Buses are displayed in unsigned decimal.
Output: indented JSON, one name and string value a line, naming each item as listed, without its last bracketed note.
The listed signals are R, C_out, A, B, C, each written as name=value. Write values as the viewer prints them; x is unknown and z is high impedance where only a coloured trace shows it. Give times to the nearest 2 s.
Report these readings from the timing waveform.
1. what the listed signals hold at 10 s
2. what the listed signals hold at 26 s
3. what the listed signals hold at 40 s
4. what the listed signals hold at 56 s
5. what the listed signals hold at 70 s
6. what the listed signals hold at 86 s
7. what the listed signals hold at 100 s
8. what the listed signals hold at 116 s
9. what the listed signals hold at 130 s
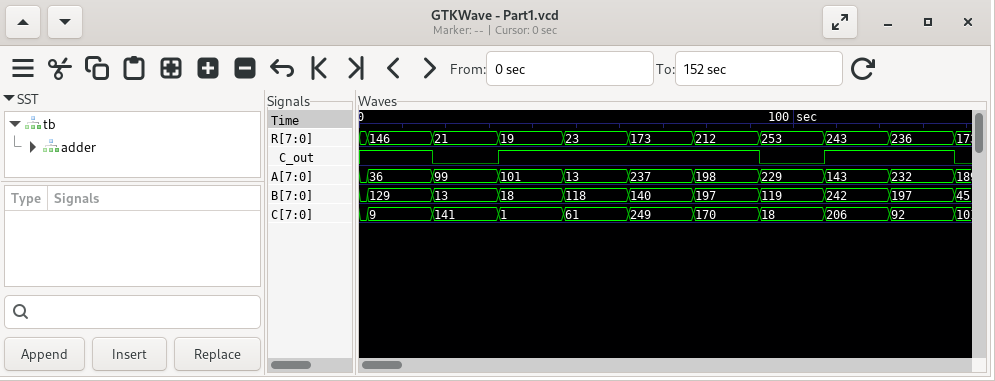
{
  "what the listed signals hold at 10 s": "R=146, C_out=1, A=36, B=129, C=9",
  "what the listed signals hold at 26 s": "R=21, C_out=0, A=99, B=13, C=141",
  "what the listed signals hold at 40 s": "R=19, C_out=1, A=101, B=18, C=1",
  "what the listed signals hold at 56 s": "R=23, C_out=1, A=13, B=118, C=61",
  "what the listed signals hold at 70 s": "R=173, C_out=1, A=237, B=140, C=249",
  "what the listed signals hold at 86 s": "R=212, C_out=1, A=198, B=197, C=170",
  "what the listed signals hold at 100 s": "R=253, C_out=0, A=229, B=119, C=18",
  "what the listed signals hold at 116 s": "R=243, C_out=1, A=143, B=242, C=206",
  "what the listed signals hold at 130 s": "R=236, C_out=1, A=232, B=197, C=92"
}
